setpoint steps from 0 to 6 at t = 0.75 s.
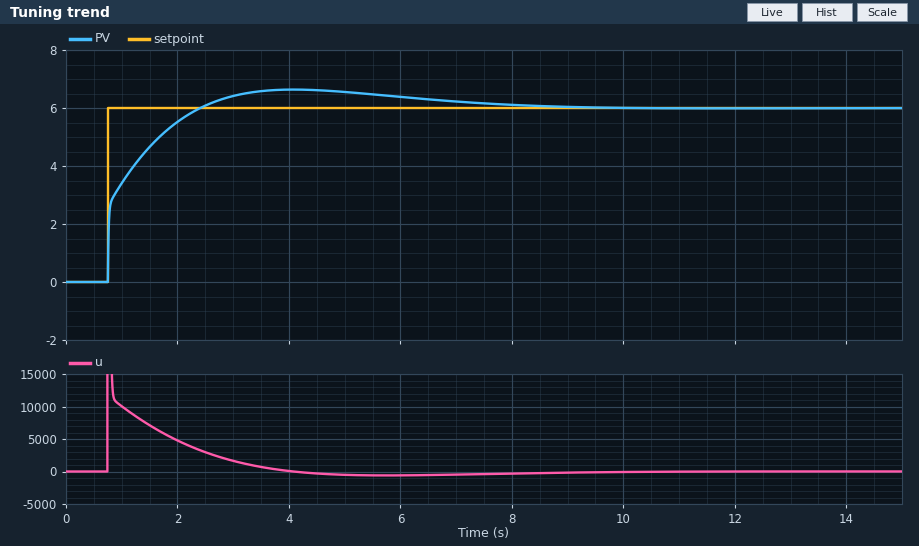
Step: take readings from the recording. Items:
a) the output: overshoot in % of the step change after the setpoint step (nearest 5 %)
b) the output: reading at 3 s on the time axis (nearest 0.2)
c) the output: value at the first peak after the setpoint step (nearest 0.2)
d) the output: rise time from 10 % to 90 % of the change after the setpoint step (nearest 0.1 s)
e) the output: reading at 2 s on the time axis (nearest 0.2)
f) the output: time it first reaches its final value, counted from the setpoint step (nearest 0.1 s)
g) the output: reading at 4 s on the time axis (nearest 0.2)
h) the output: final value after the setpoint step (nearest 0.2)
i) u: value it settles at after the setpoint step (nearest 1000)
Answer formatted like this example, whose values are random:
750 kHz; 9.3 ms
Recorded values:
10 %; 6.4; 6.6; 1.2 s; 5.6; 1.7 s; 6.6; 6.0; 0
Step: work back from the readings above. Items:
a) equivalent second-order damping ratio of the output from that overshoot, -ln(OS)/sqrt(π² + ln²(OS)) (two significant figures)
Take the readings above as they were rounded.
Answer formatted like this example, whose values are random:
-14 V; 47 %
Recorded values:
0.59
